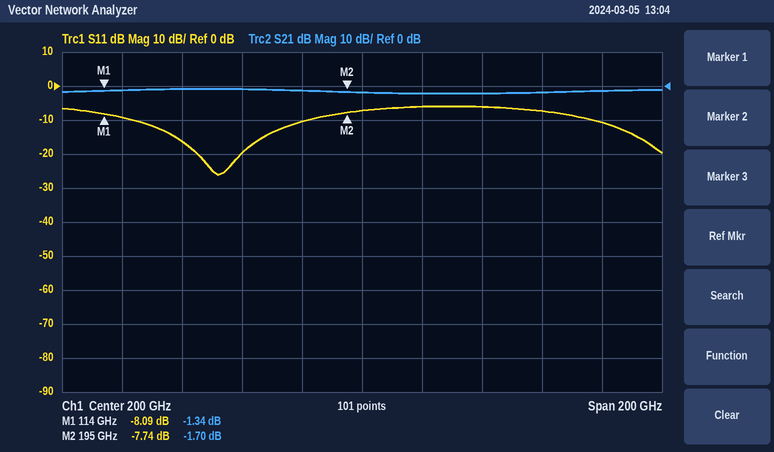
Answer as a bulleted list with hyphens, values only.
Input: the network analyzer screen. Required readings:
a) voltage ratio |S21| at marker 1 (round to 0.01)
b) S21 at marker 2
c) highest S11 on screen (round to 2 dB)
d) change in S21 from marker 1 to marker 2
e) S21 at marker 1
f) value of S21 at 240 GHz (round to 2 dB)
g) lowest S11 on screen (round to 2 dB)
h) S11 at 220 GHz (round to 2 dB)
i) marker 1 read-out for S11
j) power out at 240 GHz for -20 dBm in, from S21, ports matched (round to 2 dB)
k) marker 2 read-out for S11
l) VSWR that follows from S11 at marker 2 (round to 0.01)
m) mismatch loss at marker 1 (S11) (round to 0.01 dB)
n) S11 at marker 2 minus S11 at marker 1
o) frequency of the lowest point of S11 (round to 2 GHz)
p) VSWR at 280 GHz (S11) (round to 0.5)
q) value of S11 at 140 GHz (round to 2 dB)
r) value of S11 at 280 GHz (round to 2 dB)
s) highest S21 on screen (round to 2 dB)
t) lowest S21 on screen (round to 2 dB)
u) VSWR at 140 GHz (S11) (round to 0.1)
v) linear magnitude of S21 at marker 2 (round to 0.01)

- 0.86
- -1.70 dB
- -6 dB
- -0.36 dB
- -1.34 dB
- -2 dB
- -26 dB
- -6 dB
- -8.09 dB
- -22 dBm
- -7.74 dB
- 2.39
- 0.73 dB
- 0.35 dB
- 152 GHz
- 2.0
- -16 dB
- -10 dB
- 0 dB
- -2 dB
- 1.4
- 0.82
